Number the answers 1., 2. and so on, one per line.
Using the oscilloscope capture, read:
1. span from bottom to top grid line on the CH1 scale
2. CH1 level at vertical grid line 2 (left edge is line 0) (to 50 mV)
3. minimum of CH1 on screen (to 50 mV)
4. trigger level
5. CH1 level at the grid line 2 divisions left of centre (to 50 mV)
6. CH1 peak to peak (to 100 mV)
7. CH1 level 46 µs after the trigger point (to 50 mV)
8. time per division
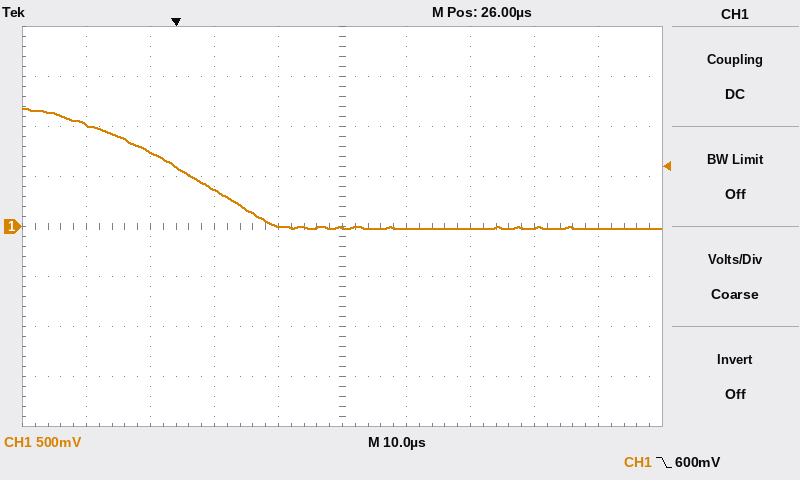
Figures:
1. 4 V
2. 750 mV
3. 0 mV
4. 600 mV
5. 350 mV
6. 1.20 V
7. 0 mV
8. 10 µs
